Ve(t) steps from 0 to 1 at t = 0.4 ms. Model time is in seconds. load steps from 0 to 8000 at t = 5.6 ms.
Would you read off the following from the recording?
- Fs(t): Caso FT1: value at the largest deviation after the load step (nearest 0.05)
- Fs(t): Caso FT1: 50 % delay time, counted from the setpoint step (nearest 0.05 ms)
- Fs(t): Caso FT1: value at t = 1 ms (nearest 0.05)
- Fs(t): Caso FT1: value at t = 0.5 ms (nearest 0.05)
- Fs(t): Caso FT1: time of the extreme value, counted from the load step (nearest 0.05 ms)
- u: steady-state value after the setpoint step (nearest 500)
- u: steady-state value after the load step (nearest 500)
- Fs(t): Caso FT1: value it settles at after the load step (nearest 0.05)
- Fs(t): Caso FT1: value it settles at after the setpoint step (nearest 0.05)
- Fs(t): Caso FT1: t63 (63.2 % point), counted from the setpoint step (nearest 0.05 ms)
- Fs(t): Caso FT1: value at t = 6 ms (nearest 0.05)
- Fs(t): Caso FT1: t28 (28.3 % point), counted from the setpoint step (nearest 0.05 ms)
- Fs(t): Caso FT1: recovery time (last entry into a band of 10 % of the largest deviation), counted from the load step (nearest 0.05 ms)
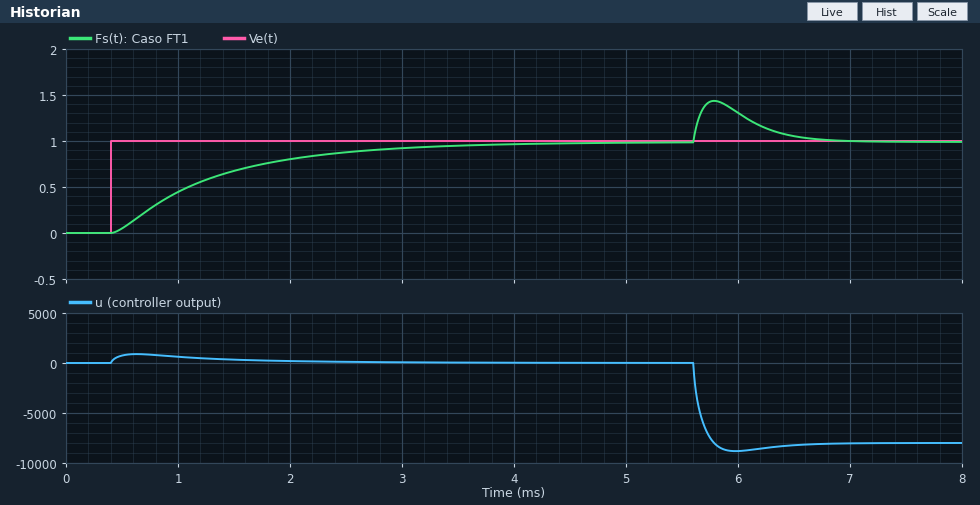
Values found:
1.45
0.70 ms
0.45
0.05
0.20 ms
0
-8000
1.00
1.00
0.95 ms
1.30
0.35 ms
1.00 ms
